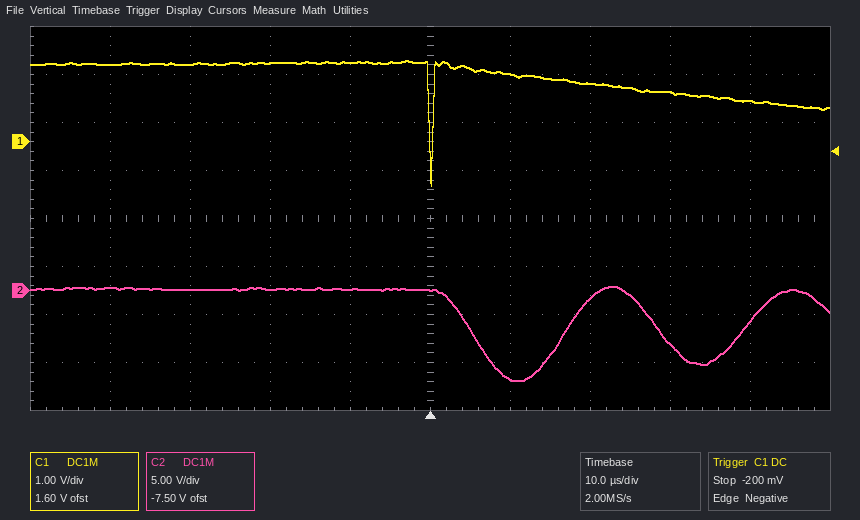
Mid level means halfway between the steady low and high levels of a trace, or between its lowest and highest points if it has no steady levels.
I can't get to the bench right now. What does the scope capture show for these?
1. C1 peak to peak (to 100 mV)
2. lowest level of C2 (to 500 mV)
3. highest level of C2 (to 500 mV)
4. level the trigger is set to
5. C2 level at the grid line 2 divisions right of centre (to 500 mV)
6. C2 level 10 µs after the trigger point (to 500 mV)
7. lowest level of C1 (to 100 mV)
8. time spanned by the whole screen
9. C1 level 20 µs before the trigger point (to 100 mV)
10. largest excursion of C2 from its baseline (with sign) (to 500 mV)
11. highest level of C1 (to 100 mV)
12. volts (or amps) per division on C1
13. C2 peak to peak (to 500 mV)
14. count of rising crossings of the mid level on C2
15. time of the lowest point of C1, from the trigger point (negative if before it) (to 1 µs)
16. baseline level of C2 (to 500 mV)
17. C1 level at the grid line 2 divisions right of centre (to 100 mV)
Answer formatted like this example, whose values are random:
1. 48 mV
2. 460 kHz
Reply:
1. 2.6 V
2. -9.5 V
3. 500 mV
4. -200 mV
5. -1.0 V
6. -9.0 V
7. -900 mV
8. 100 µs
9. 1.6 V
10. -9.5 V
11. 1.7 V
12. 1 V
13. 10.0 V
14. 2
15. 0 µs
16. 0.0 V
17. 1.2 V
